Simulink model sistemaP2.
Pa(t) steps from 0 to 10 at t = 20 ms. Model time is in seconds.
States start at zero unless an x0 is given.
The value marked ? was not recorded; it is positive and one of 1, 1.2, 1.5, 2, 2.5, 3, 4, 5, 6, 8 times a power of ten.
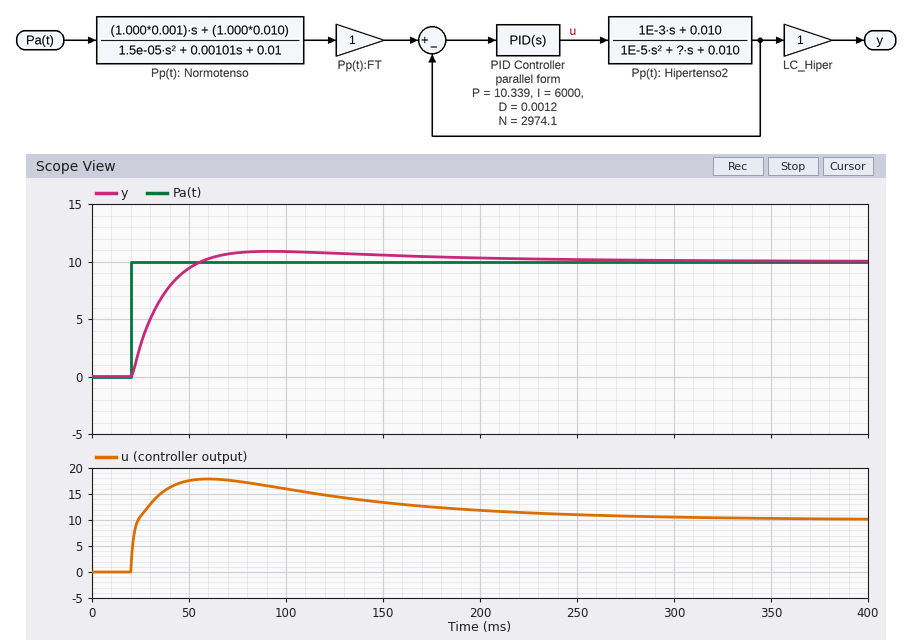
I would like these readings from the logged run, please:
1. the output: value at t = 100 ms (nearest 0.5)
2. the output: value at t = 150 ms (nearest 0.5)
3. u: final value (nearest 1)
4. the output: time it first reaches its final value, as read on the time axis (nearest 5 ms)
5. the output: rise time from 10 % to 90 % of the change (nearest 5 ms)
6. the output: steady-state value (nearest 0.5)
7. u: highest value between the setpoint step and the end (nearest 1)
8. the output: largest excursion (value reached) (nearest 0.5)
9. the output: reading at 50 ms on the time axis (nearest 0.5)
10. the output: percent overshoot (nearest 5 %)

11.0
10.5
10
55 ms
25 ms
10.0
18
11.0
9.5
10 %
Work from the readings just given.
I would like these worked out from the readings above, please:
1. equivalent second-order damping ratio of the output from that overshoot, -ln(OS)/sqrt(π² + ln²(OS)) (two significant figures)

0.59
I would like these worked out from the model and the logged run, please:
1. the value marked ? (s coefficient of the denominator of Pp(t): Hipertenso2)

0.002
